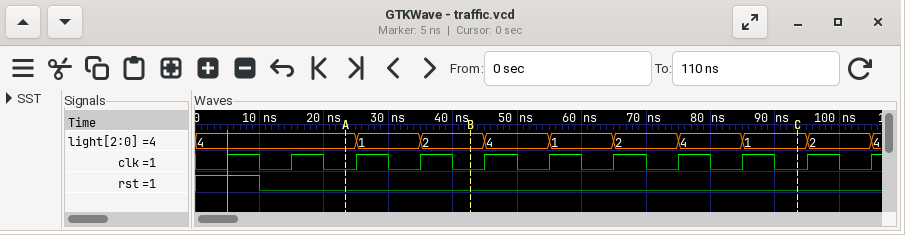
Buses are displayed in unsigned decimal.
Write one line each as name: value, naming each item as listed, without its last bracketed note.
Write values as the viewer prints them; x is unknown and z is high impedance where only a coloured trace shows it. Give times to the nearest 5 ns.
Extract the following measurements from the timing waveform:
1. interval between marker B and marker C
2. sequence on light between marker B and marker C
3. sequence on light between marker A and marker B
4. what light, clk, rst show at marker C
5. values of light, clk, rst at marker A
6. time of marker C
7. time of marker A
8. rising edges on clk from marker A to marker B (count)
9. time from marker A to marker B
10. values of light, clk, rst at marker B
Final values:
interval between marker B and marker C: 50 ns
sequence on light between marker B and marker C: 2, 4, 1, 2, 4, 1
sequence on light between marker A and marker B: 4, 1, 2
what light, clk, rst show at marker C: light=1, clk=0, rst=0
values of light, clk, rst at marker A: light=4, clk=0, rst=0
time of marker C: 95 ns
time of marker A: 25 ns
rising edges on clk from marker A to marker B: 2
time from marker A to marker B: 20 ns
values of light, clk, rst at marker B: light=2, clk=0, rst=0
